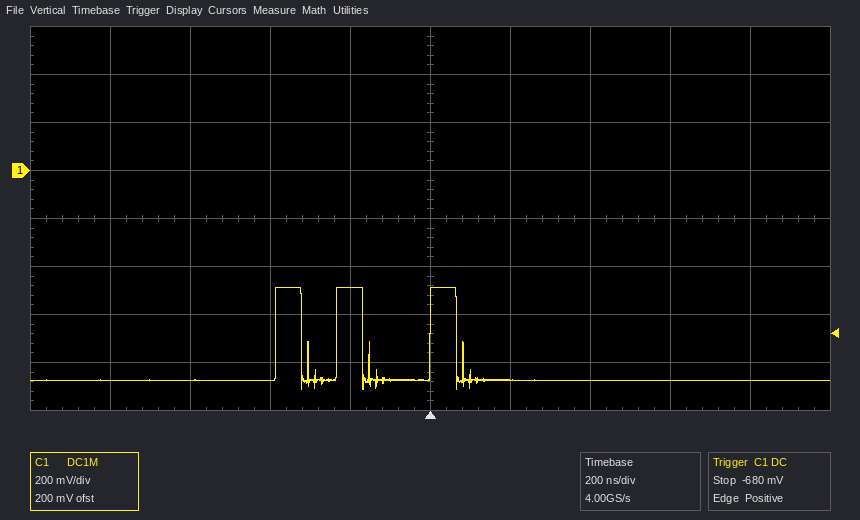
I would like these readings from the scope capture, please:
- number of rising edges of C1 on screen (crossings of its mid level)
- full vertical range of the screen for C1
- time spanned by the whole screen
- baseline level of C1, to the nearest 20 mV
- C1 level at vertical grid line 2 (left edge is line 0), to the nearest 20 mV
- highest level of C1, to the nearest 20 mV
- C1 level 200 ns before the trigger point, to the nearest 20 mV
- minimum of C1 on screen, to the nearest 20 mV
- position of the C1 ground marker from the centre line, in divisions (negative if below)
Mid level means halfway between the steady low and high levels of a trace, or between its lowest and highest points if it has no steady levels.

3
1.6 V
2 µs
-880 mV
-880 mV
-480 mV
-480 mV
-920 mV
+1.0 div
